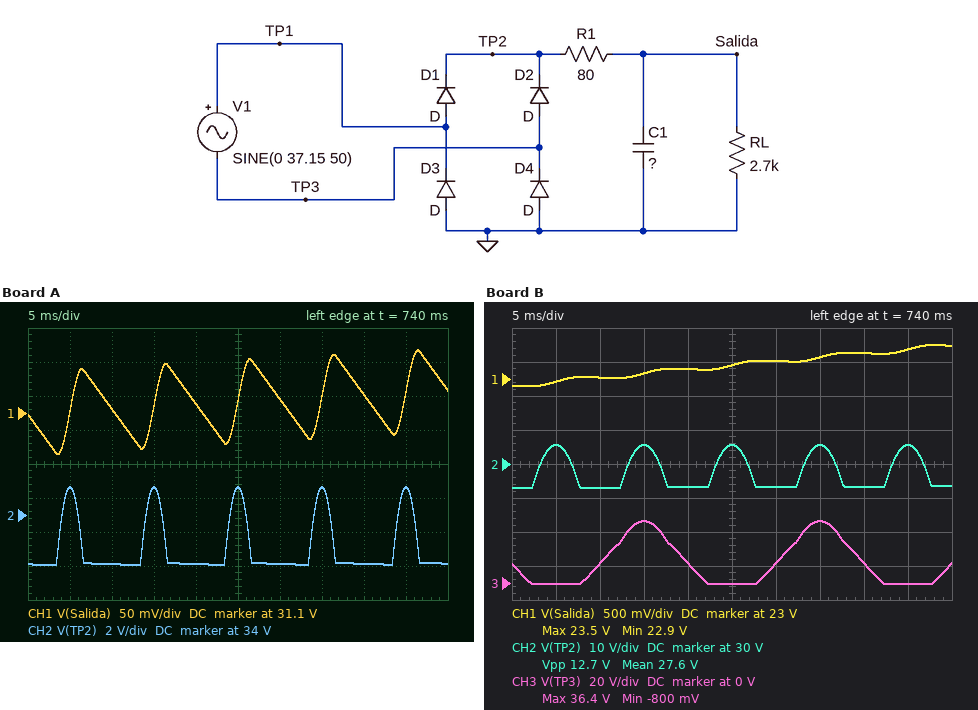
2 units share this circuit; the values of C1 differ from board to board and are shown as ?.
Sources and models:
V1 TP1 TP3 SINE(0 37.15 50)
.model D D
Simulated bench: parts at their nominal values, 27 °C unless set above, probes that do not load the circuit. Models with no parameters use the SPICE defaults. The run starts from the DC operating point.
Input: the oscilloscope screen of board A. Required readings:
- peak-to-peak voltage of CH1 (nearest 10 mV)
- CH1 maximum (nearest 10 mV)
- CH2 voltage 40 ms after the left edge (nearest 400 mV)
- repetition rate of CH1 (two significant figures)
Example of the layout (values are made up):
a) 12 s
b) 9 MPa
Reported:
a) 150 mV
b) 31.19 V
c) 31.2 V
d) 100 Hz
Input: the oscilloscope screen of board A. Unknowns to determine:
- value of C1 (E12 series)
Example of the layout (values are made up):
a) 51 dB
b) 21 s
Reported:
a) 680 µF
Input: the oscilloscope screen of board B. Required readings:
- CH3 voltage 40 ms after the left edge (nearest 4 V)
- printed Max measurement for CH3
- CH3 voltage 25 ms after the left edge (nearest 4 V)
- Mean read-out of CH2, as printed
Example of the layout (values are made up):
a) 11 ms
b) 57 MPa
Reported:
a) 12 V
b) 36.4 V
c) 0 V
d) 27.6 V
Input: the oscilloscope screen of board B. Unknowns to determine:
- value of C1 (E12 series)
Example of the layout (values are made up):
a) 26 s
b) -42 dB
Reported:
a) 3.9 mF
